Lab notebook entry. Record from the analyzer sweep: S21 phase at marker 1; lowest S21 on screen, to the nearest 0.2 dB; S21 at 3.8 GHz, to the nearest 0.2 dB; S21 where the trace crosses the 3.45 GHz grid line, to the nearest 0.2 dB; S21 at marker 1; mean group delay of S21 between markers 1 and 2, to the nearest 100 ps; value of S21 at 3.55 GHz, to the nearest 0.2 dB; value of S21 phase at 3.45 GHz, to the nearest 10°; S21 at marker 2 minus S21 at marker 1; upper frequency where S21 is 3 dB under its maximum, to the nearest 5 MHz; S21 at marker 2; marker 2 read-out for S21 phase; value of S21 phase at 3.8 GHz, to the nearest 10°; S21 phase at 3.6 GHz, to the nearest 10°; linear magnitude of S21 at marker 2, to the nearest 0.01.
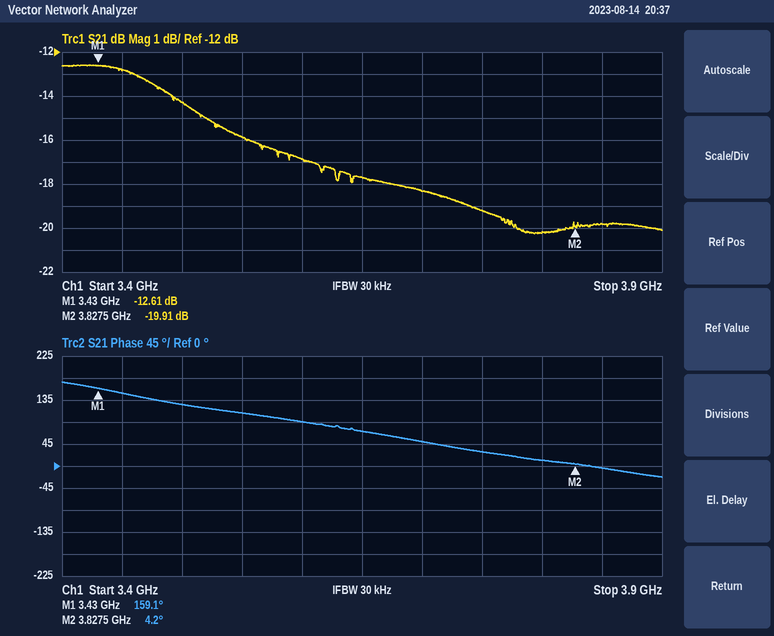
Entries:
159.1°
-20.2 dB
-20.2 dB
-12.8 dB
-12.61 dB
1.1 ns
-15.8 dB
150°
-7.30 dB
3.540 GHz
-19.91 dB
4.2°
10°
90°
0.10
